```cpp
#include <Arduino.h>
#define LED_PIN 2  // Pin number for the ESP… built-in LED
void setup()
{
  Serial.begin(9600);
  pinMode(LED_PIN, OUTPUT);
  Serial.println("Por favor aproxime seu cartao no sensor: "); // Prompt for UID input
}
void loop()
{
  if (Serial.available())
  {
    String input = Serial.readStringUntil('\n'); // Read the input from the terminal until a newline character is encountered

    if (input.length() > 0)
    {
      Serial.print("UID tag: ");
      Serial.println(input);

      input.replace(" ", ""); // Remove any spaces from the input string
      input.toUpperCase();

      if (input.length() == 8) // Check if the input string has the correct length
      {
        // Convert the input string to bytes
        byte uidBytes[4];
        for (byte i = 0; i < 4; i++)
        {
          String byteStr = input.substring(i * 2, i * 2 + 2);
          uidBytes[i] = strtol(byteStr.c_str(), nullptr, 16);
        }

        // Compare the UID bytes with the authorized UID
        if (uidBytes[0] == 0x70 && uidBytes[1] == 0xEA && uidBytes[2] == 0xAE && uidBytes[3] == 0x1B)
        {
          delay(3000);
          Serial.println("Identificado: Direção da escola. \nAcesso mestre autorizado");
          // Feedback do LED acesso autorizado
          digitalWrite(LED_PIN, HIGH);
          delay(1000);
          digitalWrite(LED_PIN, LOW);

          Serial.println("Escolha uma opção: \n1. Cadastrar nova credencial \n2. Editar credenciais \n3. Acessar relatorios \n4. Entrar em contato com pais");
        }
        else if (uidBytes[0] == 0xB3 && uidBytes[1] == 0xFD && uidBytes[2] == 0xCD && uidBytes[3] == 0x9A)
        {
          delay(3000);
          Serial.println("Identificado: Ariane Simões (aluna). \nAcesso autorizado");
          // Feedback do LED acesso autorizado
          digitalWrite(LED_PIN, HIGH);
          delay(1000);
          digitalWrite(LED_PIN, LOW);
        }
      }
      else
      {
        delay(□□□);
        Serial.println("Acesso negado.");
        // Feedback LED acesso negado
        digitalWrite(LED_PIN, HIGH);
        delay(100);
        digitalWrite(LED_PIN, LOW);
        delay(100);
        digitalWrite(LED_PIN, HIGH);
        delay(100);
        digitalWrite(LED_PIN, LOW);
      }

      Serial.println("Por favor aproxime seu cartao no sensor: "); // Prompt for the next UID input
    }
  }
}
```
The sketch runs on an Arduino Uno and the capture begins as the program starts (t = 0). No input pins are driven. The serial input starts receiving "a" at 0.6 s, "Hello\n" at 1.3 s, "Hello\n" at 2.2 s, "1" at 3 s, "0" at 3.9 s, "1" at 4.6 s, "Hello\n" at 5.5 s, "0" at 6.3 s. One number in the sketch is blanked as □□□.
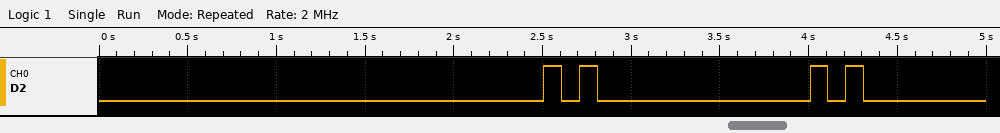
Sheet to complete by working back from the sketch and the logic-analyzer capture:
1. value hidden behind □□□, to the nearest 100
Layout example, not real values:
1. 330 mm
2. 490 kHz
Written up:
1. 1200
